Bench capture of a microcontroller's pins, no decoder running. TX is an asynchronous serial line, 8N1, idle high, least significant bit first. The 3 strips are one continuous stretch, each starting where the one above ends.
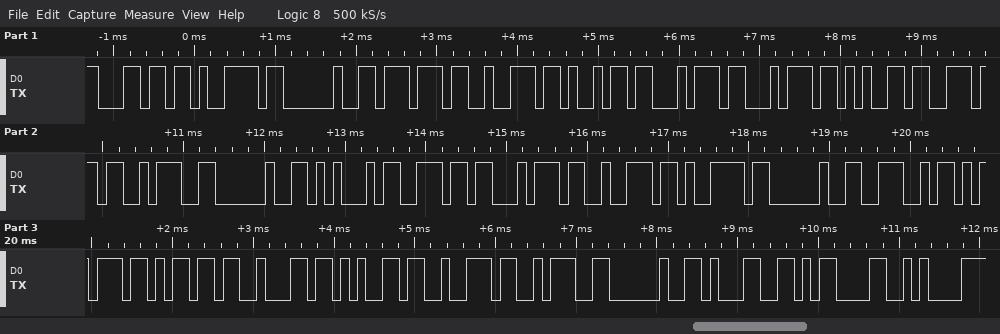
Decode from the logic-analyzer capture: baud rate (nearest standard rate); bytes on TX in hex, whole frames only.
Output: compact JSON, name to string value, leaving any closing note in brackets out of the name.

{"baud rate": "9600 baud", "bytes on TX in hex, whole frames only": "6C 79 20 77 72 69 74 74 65 6E 3A 20 45 6E 74 72 79 20 4E 75 6D 62 65 72 3A 20 31 0D 0A"}
